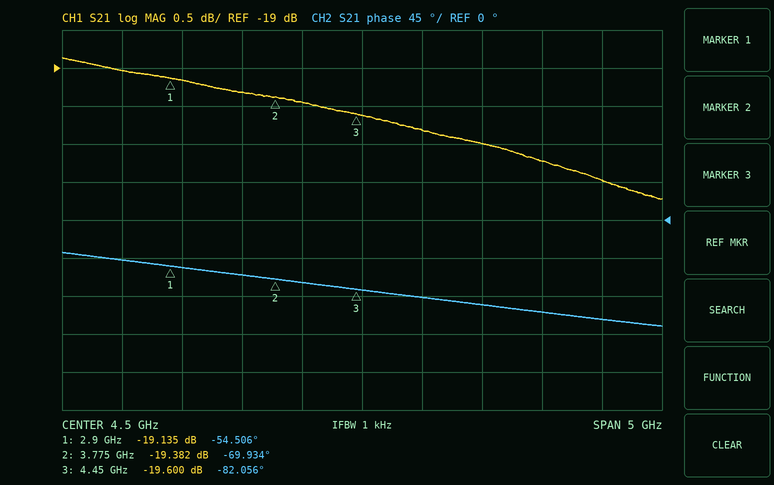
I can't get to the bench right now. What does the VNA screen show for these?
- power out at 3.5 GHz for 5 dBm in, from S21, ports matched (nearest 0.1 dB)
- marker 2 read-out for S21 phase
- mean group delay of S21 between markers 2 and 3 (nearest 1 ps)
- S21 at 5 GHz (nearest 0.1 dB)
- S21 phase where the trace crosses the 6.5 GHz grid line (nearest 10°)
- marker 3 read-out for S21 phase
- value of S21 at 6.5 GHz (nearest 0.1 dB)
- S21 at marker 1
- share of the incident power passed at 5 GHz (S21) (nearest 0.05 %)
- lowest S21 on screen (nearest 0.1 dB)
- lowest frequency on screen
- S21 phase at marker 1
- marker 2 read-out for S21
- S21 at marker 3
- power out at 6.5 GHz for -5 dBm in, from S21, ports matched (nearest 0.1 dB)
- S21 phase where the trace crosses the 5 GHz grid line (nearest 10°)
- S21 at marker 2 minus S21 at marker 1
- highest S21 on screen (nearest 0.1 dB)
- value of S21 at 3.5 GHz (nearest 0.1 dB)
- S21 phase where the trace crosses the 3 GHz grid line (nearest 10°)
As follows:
-14.3 dBm
-69.934°
50 ps
-19.8 dB
-120°
-82.056°
-20.5 dB
-19.135 dB
1.05 %
-20.7 dB
2 GHz
-54.506°
-19.382 dB
-19.600 dB
-25.5 dBm
-90°
-0.247 dB
-18.9 dB
-19.3 dB
-60°
